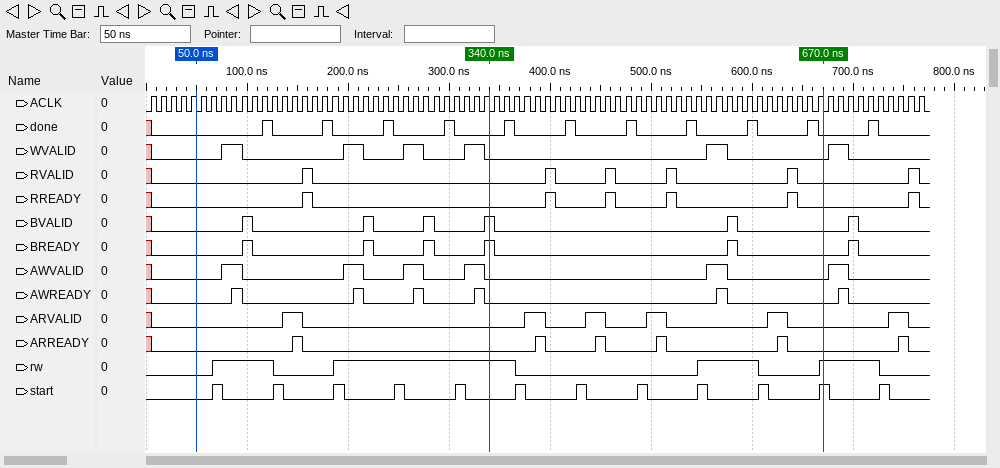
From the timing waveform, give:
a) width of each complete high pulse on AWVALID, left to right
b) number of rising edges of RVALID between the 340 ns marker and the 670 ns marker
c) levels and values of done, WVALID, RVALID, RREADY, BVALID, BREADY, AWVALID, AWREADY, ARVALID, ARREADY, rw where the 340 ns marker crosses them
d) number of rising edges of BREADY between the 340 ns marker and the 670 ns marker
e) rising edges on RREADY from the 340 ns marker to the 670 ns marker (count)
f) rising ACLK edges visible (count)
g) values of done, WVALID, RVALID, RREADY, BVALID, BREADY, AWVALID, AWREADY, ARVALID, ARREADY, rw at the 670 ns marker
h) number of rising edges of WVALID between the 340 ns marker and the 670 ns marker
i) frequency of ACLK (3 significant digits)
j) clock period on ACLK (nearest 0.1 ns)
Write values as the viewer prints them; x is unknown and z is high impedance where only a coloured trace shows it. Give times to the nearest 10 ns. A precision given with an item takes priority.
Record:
20 ns, 20 ns, 20 ns, 20 ns, 20 ns, 20 ns
4
done=0, WVALID=0, RVALID=0, RREADY=0, BVALID=1, BREADY=1, AWVALID=0, AWREADY=0, ARVALID=0, ARREADY=0, rw=1
1
4
77
done=0, WVALID=0, RVALID=0, RREADY=0, BVALID=0, BREADY=0, AWVALID=0, AWREADY=0, ARVALID=0, ARREADY=0, rw=1
1
100 MHz
10 ns
